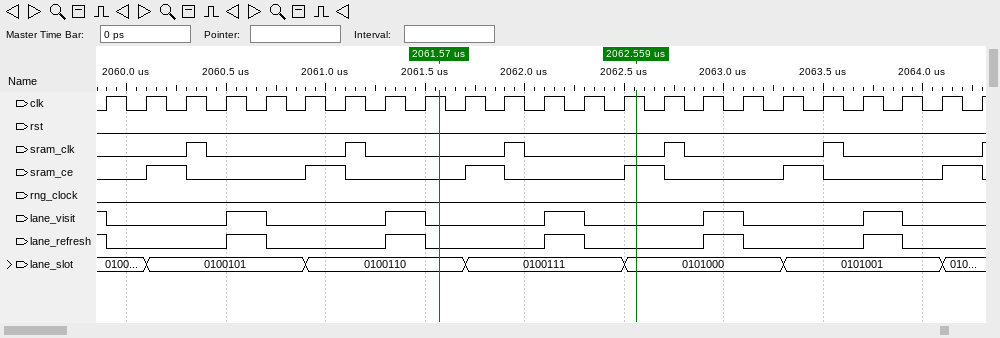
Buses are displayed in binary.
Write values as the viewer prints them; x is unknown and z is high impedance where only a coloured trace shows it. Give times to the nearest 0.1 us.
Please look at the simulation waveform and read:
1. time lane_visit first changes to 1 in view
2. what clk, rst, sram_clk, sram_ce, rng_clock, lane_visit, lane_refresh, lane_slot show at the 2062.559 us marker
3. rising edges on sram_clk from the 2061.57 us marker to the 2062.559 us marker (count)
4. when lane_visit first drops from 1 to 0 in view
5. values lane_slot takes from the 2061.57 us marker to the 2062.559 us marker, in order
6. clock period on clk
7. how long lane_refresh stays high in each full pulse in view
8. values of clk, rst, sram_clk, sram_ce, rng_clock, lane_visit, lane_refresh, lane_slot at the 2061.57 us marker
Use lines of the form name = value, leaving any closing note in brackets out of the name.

time lane_visit first changes to 1 in view = 2060.5 us
what clk, rst, sram_clk, sram_ce, rng_clock, lane_visit, lane_refresh, lane_slot show at the 2062.559 us marker = clk=1, rst=0, sram_clk=0, sram_ce=1, rng_clock=0, lane_visit=0, lane_refresh=0, lane_slot=0101000
rising edges on sram_clk from the 2061.57 us marker to the 2062.559 us marker = 1
when lane_visit first drops from 1 to 0 in view = 2059.9 us
values lane_slot takes from the 2061.57 us marker to the 2062.559 us marker, in order = 0100110, 0100111, 0101000
clock period on clk = 0.2 us
how long lane_refresh stays high in each full pulse in view = 0.2 us, 0.2 us, 0.2 us, 0.2 us, 0.2 us
values of clk, rst, sram_clk, sram_ce, rng_clock, lane_visit, lane_refresh, lane_slot at the 2061.57 us marker = clk=1, rst=0, sram_clk=0, sram_ce=0, rng_clock=0, lane_visit=0, lane_refresh=0, lane_slot=0100110
